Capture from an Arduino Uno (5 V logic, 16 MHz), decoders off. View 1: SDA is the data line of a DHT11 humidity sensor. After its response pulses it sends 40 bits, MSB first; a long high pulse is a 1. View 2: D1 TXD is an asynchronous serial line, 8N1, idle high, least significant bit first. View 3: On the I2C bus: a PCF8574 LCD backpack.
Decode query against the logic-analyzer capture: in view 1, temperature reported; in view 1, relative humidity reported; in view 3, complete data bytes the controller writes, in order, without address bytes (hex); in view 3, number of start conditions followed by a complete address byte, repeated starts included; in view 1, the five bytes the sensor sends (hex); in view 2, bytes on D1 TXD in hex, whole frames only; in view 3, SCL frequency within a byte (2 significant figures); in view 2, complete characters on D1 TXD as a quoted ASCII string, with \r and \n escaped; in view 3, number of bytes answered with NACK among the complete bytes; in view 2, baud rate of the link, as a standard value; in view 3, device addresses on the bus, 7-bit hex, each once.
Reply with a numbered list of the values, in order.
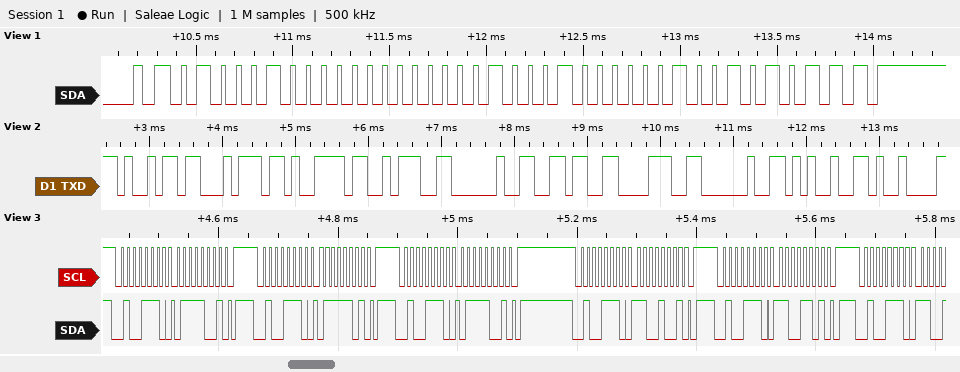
1. 17.2 °C
2. 68 %
3. 79 7D 79 C9 CD
4. 6
5. 44 00 11 02 57
6. 69 74 79 3A 20 36 38 20 25 09
7. 100 kHz
8. "ity: 68 %\t"
9. 0
10. 9600 baud
11. 0x27
